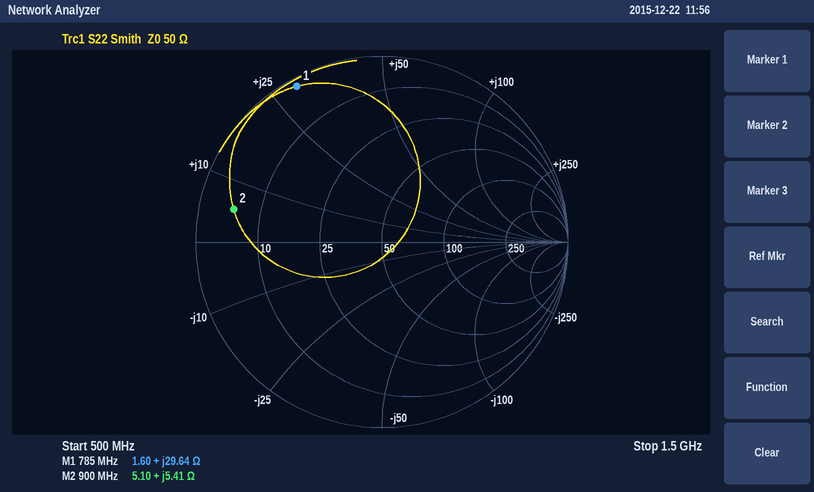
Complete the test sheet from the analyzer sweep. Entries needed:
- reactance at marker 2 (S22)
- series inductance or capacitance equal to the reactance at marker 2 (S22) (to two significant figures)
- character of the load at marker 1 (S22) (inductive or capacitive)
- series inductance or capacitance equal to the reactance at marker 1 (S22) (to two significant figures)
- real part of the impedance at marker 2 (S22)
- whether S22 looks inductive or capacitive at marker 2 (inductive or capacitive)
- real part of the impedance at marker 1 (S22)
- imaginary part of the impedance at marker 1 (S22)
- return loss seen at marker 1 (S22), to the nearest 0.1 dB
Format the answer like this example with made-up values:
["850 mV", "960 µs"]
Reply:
["+5.41 Ω", "960 pH", "inductive", "6.0 nH", "5.10 Ω", "inductive", "1.60 Ω", "+29.64 Ω", "0.4 dB"]
